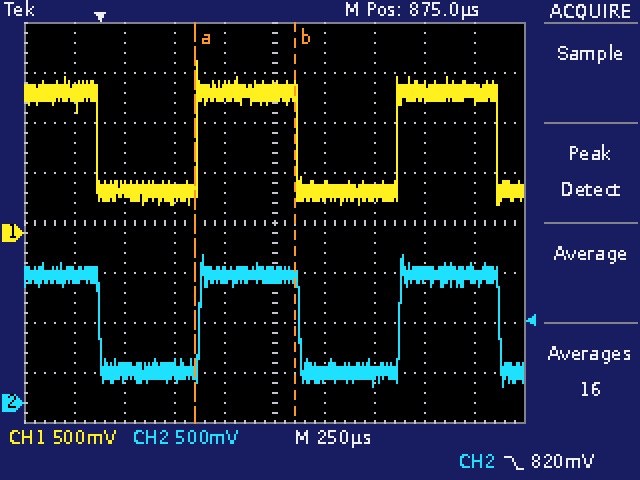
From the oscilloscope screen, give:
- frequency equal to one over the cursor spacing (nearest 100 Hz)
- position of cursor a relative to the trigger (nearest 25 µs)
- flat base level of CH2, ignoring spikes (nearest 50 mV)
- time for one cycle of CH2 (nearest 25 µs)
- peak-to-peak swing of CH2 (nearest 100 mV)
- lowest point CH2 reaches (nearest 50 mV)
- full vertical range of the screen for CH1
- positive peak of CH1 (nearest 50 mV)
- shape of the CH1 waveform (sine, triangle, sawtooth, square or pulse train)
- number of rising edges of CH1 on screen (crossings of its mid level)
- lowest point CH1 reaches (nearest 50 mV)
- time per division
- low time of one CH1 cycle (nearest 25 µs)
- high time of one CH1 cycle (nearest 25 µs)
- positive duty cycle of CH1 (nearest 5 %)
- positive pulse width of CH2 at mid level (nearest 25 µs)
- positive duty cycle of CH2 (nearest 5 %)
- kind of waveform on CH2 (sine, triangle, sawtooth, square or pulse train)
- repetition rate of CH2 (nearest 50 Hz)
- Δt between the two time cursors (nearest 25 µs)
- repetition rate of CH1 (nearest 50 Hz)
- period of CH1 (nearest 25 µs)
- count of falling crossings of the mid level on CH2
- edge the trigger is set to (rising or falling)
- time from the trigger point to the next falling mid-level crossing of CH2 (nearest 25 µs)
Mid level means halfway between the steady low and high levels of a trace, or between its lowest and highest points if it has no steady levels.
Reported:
2.0 kHz
+475 µs
300 mV
1.000 ms
1.30 V
150 mV
4 V
1.70 V
square
2
300 mV
250 µs
500 µs
500 µs
50 %
500 µs
50 %
square
1.00 kHz
500 µs
1.00 kHz
1.000 ms
3
falling
1.000 ms
